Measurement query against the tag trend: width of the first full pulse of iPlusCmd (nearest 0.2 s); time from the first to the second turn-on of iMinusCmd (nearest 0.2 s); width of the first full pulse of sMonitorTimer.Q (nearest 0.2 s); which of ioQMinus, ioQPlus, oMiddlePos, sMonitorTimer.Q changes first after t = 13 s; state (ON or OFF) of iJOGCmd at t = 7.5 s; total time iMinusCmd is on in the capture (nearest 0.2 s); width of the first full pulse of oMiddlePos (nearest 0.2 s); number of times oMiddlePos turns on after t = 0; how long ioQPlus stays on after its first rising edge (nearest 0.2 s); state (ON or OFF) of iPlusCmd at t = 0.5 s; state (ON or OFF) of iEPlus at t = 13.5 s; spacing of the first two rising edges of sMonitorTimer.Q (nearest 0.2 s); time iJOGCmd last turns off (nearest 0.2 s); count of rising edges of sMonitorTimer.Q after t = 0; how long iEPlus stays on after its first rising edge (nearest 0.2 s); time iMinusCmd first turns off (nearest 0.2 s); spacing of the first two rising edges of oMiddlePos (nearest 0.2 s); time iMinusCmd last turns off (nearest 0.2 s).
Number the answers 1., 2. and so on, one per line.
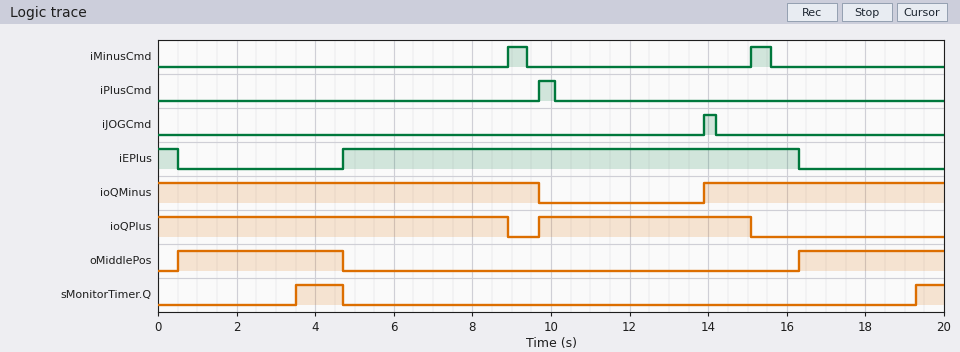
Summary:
1. 0.4 s
2. 6.2 s
3. 1.2 s
4. ioQMinus
5. OFF
6. 1.0 s
7. 4.2 s
8. 2
9. 5.4 s
10. OFF
11. ON
12. 15.8 s
13. 14.2 s
14. 2
15. 11.6 s
16. 9.4 s
17. 15.8 s
18. 15.6 s
